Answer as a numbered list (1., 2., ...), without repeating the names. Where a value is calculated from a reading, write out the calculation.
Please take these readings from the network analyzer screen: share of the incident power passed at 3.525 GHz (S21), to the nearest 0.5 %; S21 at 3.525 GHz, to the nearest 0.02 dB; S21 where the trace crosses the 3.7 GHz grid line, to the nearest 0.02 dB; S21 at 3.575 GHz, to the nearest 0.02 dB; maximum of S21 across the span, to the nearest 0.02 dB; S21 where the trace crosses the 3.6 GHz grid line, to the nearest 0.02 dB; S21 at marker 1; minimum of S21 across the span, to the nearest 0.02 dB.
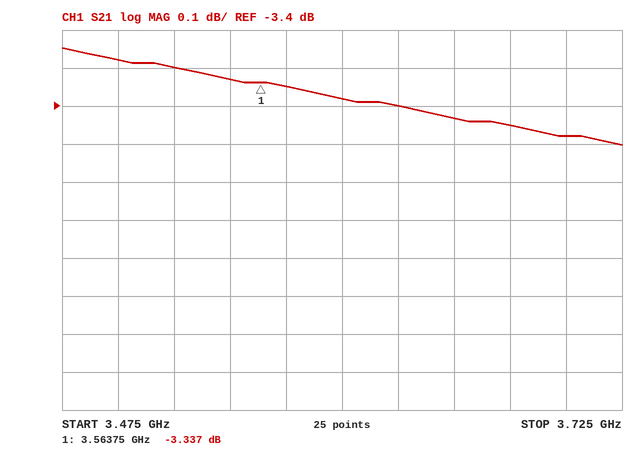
1. 10^(-3.3/10) ≈ 46.8 %, so 47.0 % to the nearest 0.5 %
2. -3.30 dB
3. -3.48 dB
4. -3.34 dB
5. -3.24 dB
6. -3.38 dB
7. -3.337 dB
8. -3.50 dB
